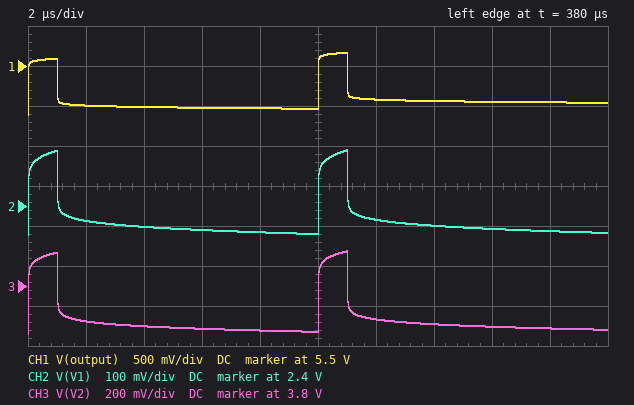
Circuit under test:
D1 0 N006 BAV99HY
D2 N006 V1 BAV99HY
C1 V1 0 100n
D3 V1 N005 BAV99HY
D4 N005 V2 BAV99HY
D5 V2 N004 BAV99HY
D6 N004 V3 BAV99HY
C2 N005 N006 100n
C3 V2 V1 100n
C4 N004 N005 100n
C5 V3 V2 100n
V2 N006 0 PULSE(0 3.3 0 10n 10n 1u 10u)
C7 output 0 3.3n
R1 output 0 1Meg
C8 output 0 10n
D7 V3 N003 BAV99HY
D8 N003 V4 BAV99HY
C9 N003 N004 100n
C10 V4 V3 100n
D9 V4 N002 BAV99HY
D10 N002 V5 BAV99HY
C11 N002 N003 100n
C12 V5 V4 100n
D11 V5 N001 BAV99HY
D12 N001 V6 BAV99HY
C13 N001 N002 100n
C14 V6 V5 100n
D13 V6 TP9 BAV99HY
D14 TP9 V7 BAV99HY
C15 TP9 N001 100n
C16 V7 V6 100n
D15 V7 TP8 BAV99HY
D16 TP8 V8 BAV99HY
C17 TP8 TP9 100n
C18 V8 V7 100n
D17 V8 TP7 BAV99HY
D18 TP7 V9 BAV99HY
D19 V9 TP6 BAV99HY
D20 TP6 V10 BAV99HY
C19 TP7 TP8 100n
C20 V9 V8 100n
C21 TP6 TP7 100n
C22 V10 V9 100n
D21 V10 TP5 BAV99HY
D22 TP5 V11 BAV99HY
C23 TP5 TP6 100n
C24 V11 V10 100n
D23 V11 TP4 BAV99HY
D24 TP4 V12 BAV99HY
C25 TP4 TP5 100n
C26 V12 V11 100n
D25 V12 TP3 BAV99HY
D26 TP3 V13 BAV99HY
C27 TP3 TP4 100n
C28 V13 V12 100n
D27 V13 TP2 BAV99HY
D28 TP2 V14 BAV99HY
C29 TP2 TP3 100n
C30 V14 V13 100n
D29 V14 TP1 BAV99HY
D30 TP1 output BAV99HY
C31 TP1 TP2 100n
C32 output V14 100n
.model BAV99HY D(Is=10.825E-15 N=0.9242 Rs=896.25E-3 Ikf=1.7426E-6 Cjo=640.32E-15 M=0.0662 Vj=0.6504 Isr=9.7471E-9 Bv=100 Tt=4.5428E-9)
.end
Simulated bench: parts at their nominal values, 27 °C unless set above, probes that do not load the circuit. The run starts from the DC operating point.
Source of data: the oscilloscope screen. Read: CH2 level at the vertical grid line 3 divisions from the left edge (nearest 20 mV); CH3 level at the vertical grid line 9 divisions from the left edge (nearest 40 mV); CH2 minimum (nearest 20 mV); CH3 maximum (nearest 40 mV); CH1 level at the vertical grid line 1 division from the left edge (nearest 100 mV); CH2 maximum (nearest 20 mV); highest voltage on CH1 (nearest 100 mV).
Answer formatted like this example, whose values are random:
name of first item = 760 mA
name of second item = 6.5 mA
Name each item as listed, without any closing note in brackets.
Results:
CH2 level at the vertical grid line 3 divisions from the left edge = 2.34 V
CH3 level at the vertical grid line 9 divisions from the left edge = 3.60 V
CH2 minimum = 2.32 V
CH3 maximum = 3.96 V
CH1 level at the vertical grid line 1 division from the left edge = 5.0 V
CH2 maximum = 2.54 V
highest voltage on CH1 = 5.7 V
